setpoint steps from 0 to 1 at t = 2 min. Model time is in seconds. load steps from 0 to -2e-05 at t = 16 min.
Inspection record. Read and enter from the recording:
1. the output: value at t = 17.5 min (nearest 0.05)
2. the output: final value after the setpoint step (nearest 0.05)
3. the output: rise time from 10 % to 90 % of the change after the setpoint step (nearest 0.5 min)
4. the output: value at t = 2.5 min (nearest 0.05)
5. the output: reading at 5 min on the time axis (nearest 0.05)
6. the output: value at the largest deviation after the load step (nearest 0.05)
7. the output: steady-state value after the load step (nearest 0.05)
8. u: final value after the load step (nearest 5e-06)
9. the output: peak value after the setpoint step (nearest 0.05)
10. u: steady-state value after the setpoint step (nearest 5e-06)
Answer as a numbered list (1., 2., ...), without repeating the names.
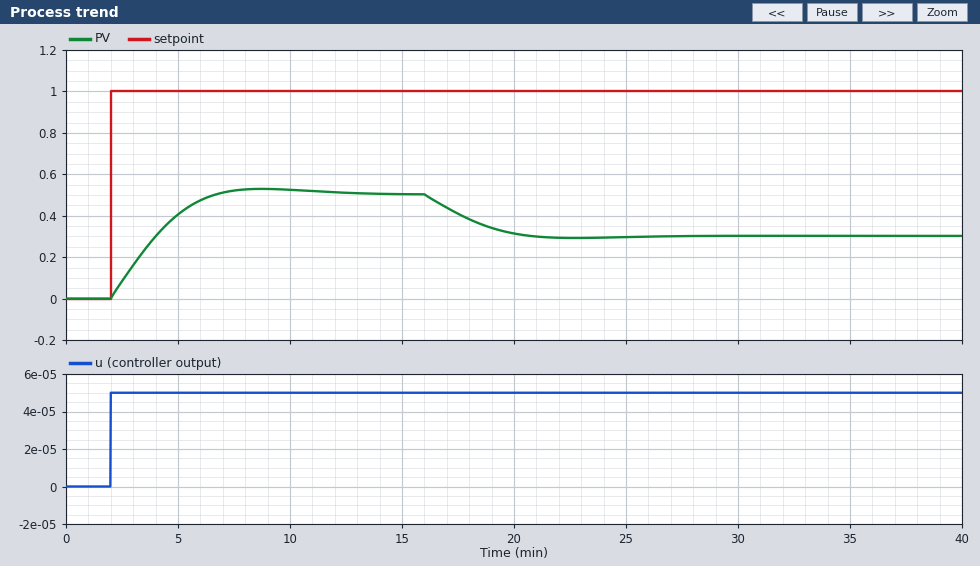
1. 0.40
2. 0.50
3. 3.5 min
4. 0.10
5. 0.40
6. 0.30
7. 0.30
8. 0.000050
9. 0.55
10. 0.000050
